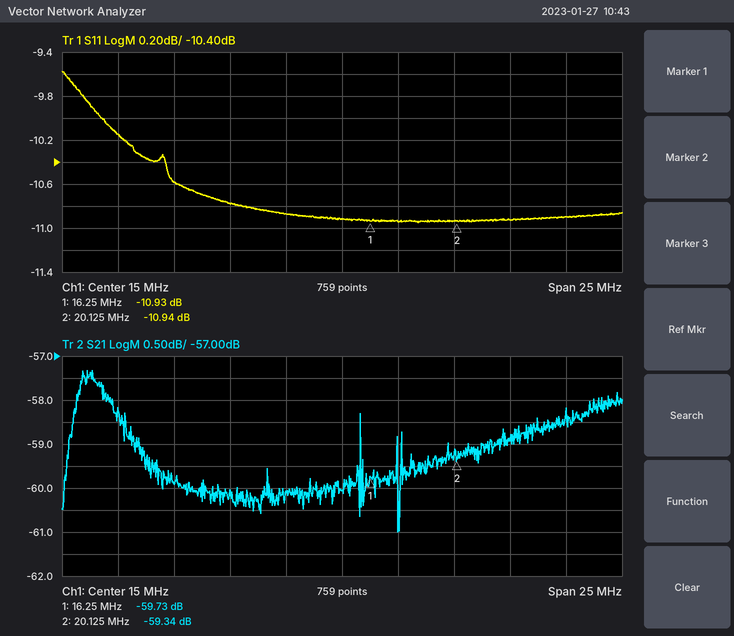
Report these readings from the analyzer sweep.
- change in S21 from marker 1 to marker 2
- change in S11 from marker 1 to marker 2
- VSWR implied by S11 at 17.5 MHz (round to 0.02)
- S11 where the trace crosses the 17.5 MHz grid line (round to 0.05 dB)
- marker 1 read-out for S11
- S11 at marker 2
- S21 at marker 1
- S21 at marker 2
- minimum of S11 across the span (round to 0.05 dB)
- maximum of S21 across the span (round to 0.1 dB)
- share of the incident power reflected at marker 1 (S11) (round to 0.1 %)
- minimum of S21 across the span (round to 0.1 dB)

0.39 dB
-0.01 dB
1.80
-10.95 dB
-10.93 dB
-10.94 dB
-59.73 dB
-59.34 dB
-10.95 dB
-57.3 dB
8.1 %
-61.0 dB
